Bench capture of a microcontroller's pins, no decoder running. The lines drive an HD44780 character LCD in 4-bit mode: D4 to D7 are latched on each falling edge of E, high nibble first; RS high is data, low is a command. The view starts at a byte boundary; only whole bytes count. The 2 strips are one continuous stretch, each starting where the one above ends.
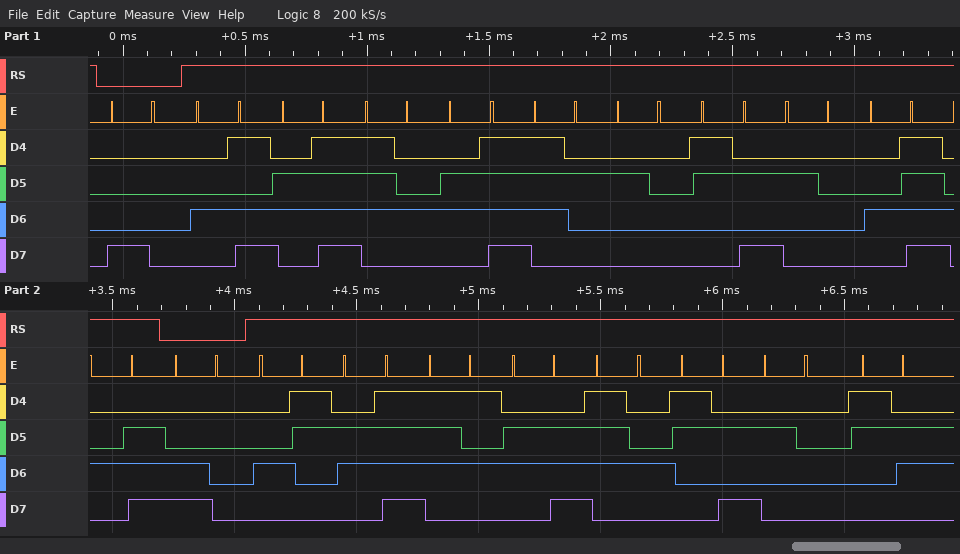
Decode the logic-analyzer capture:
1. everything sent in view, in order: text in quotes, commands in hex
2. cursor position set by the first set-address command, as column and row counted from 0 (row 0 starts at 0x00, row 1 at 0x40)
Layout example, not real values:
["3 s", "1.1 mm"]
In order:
["0x80 \"Motor : ON\" 0xC0 \"Count: 6\"", "column 0, row 0"]
